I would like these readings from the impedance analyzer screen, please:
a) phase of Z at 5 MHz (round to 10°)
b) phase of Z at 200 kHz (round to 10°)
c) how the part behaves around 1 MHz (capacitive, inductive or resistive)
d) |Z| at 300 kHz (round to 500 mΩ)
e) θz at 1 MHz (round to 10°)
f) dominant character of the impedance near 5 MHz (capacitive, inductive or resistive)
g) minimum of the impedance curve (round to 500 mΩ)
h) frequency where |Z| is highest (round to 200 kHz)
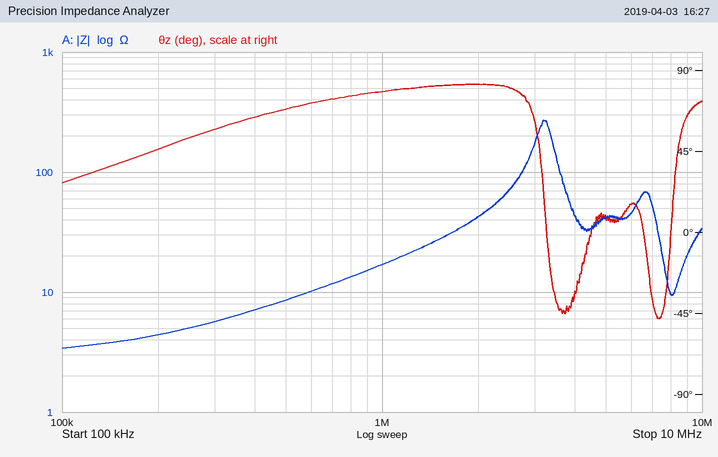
10°
50°
inductive
5.5 Ω
80°
resistive
3.5 Ω
3.2 MHz
